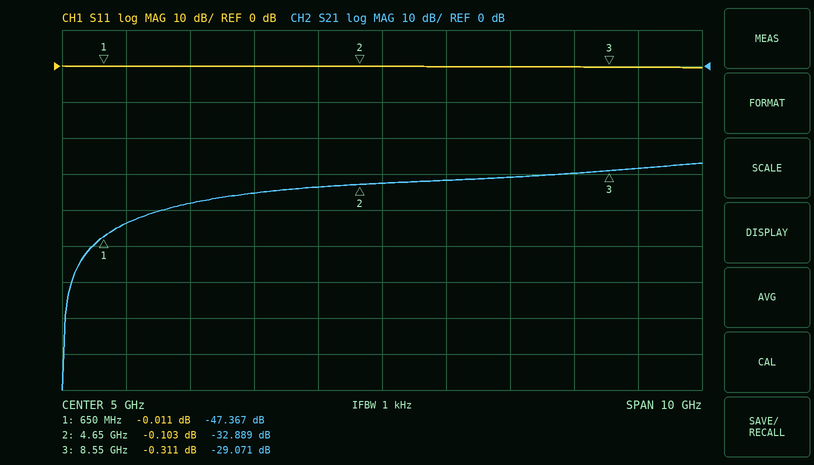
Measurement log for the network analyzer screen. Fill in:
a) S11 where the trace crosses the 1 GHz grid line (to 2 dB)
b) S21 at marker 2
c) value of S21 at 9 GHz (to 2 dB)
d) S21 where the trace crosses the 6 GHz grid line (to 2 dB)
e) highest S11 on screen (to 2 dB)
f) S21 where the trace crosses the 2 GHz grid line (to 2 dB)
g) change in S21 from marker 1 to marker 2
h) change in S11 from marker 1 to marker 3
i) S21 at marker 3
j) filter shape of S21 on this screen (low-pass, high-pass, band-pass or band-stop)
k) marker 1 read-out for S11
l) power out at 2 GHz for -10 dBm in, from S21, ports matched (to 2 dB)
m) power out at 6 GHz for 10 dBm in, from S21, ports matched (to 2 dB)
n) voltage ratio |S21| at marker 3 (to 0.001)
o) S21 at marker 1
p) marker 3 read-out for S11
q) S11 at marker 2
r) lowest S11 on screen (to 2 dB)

0 dB
-32.889 dB
-28 dB
-32 dB
0 dB
-38 dB
14.478 dB
-0.300 dB
-29.071 dB
high-pass
-0.011 dB
-48 dBm
-22 dBm
0.035
-47.367 dB
-0.311 dB
-0.103 dB
0 dB
